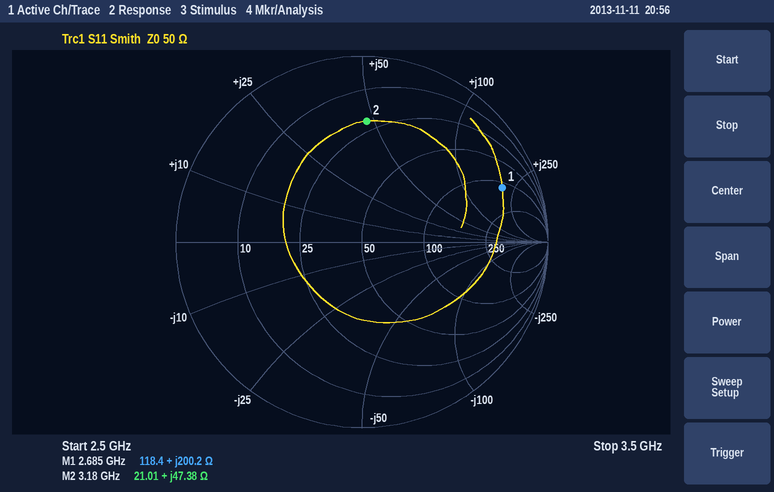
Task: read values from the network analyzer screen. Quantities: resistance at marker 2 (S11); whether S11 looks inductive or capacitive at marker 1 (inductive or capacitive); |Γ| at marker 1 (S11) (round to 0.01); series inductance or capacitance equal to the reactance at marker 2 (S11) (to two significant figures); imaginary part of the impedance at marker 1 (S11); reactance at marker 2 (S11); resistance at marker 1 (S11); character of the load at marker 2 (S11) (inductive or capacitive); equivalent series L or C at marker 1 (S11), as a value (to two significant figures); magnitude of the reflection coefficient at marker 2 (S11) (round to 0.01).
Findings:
21.01 Ω
inductive
0.81
2.4 nH
+200.2 Ω
+47.38 Ω
118.4 Ω
inductive
12 nH
0.65
